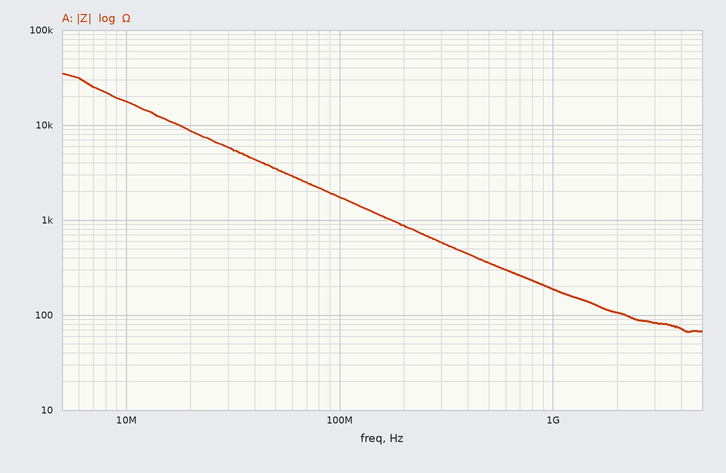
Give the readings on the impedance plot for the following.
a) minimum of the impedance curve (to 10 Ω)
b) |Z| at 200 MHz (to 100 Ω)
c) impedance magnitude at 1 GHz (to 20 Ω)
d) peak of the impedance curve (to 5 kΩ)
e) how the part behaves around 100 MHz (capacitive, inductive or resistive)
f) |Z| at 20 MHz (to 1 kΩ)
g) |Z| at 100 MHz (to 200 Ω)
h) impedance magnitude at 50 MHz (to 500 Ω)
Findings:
70 Ω
900 Ω
180 Ω
35 kΩ
capacitive
9 kΩ
1.8 kΩ
3.5 kΩ
